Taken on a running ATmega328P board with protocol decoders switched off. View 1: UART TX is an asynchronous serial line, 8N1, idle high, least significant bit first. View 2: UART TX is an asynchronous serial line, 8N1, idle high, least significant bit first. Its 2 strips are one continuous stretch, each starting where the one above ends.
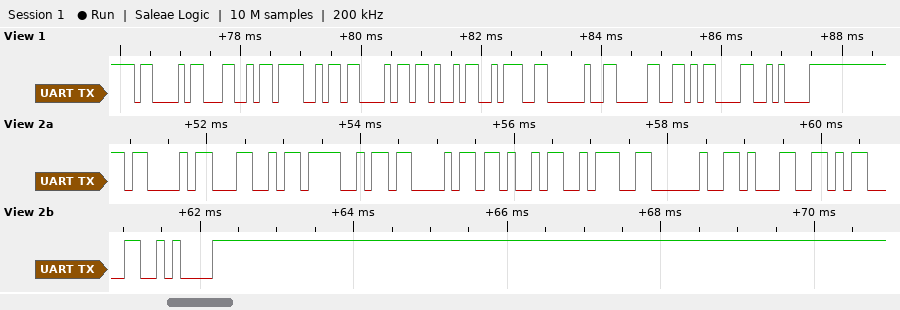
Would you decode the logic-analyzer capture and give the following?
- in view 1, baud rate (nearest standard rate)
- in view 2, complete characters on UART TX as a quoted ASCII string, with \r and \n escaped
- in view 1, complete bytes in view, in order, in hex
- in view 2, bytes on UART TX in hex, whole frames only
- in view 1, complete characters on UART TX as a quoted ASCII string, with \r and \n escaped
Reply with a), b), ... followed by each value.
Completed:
a) 9600 baud
b) "CLOCK: 1\r\n"
c) 43 4C 4F 43 4B 3A 20 30 0D 0A
d) 43 4C 4F 43 4B 3A 20 31 0D 0A
e) "CLOCK: 0\r\n"
